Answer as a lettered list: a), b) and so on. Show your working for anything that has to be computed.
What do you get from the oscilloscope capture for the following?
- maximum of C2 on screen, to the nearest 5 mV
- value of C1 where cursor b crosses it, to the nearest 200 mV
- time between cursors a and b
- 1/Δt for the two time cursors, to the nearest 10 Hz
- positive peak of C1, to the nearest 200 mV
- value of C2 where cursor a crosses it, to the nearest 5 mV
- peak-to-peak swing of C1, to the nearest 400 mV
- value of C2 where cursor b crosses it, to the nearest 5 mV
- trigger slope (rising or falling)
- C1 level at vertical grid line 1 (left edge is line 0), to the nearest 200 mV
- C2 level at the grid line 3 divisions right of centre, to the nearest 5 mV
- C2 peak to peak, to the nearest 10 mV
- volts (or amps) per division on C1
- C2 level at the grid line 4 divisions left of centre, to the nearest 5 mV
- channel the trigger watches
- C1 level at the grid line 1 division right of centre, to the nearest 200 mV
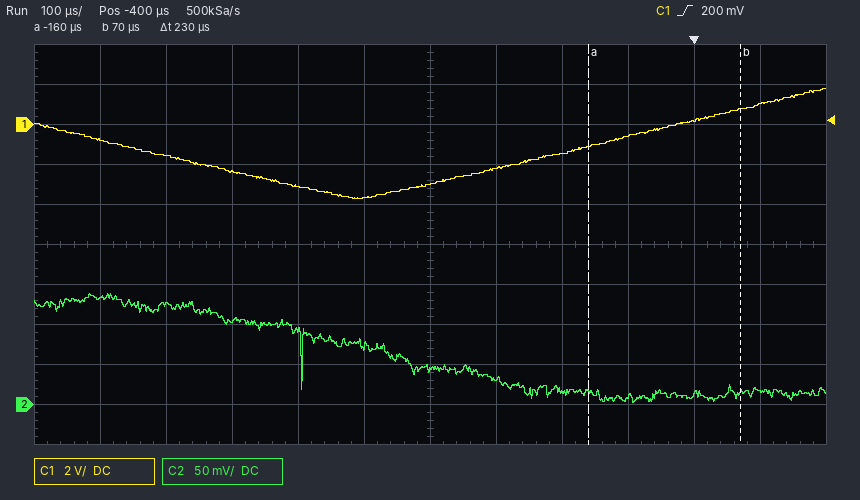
a) 140 mV
b) 800 mV
c) 230 µs
d) 1 / 230 µs ≈ 4.35 kHz
e) 1.8 V
f) 15 mV
g) 5.6 V
h) 15 mV
i) rising
j) -800 mV
k) 10 mV
l) 140 mV
m) 2 V
n) 125 mV
o) C1
p) -2.2 V
